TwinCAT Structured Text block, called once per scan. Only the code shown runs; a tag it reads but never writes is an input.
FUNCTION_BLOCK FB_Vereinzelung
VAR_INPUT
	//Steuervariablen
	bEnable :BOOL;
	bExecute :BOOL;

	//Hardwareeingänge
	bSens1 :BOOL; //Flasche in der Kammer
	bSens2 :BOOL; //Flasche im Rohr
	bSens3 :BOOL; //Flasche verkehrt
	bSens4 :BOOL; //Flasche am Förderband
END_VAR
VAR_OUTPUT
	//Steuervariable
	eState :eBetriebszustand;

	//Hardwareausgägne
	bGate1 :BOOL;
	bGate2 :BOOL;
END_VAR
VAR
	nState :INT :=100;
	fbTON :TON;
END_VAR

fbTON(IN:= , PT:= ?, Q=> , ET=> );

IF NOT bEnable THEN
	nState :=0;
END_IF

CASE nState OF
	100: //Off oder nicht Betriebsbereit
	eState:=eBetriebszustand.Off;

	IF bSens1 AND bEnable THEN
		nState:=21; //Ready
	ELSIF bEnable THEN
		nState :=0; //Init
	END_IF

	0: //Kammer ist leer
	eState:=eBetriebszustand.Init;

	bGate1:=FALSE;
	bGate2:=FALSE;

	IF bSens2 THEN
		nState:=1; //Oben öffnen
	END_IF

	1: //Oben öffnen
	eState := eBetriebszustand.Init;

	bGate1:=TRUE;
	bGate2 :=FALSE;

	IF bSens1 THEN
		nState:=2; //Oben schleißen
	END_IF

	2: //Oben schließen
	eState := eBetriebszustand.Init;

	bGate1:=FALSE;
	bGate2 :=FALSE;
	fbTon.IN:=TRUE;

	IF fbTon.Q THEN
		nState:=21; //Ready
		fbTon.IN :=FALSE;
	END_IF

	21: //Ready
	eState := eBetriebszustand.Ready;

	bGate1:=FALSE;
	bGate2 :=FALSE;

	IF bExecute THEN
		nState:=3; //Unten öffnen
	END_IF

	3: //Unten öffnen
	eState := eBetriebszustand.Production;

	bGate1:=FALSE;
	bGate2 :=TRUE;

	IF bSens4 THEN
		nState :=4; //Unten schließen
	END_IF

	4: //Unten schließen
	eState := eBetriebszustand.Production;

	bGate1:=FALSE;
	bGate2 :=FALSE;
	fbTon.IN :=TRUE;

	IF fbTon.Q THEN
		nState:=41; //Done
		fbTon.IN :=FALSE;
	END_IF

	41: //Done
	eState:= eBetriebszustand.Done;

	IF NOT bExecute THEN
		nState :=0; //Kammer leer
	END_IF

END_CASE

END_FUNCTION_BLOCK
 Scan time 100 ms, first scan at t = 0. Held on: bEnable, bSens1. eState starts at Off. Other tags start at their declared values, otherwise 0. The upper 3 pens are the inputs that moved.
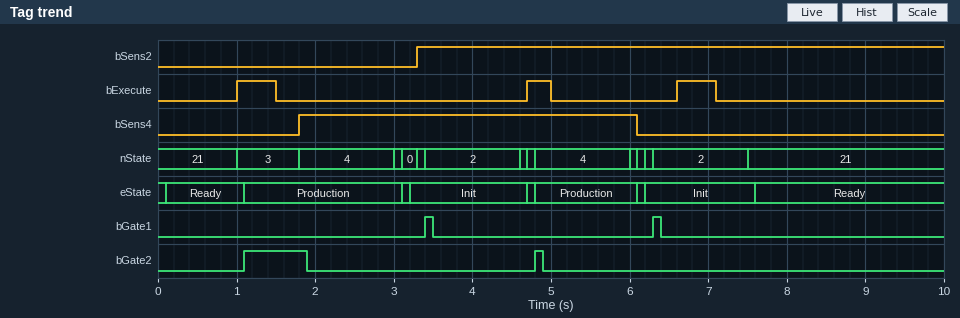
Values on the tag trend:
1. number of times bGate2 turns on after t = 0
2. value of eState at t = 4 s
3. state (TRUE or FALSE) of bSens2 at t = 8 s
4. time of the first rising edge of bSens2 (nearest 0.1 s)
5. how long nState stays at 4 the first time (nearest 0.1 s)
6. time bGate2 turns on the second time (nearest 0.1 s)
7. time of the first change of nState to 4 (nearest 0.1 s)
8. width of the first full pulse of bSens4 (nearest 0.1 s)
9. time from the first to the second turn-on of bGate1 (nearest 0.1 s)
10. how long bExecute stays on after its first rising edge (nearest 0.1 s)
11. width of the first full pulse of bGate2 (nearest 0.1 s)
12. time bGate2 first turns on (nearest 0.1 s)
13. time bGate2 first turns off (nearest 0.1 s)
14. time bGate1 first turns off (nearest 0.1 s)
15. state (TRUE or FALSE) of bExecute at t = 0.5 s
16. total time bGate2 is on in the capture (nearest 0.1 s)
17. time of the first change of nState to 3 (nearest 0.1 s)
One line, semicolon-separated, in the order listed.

2; Init; TRUE; 3.3 s; 1.2 s; 4.8 s; 1.8 s; 4.3 s; 2.9 s; 0.5 s; 0.8 s; 1.1 s; 1.9 s; 3.5 s; FALSE; 0.9 s; 1.0 s
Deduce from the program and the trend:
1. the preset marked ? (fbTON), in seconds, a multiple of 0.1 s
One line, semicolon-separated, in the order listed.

1.0 s
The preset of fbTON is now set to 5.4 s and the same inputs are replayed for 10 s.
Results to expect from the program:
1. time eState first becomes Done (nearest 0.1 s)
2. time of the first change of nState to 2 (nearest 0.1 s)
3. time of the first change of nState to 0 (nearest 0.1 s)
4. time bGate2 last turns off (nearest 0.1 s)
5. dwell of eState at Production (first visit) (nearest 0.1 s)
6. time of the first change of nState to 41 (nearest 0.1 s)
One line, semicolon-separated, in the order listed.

7.5 s; 7.7 s; 7.5 s; 1.9 s; 6.4 s; 7.4 s
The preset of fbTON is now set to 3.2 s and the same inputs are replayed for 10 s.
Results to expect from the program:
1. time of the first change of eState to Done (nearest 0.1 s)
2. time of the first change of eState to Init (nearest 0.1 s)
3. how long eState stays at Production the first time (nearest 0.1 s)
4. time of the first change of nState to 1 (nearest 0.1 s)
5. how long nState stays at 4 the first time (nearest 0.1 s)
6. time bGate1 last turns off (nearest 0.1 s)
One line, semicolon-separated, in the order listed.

5.3 s; 5.4 s; 4.2 s; 5.4 s; 3.4 s; 5.6 s
